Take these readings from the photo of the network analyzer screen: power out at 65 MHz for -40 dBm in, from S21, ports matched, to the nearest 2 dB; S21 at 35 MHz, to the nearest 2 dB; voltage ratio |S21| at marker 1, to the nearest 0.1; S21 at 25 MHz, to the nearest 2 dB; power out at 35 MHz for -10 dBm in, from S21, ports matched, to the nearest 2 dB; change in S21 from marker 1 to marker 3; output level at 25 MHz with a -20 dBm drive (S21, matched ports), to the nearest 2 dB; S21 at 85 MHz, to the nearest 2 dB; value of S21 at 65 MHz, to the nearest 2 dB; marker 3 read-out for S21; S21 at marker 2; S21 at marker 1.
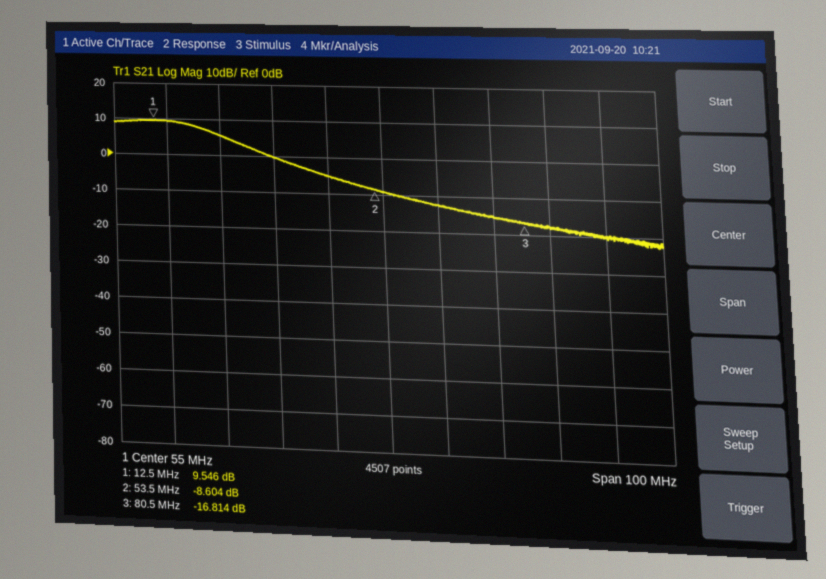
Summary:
-52 dBm
0 dB
3.0
6 dB
-10 dBm
-26.360 dB
-14 dBm
-18 dB
-12 dB
-16.814 dB
-8.604 dB
9.546 dB
